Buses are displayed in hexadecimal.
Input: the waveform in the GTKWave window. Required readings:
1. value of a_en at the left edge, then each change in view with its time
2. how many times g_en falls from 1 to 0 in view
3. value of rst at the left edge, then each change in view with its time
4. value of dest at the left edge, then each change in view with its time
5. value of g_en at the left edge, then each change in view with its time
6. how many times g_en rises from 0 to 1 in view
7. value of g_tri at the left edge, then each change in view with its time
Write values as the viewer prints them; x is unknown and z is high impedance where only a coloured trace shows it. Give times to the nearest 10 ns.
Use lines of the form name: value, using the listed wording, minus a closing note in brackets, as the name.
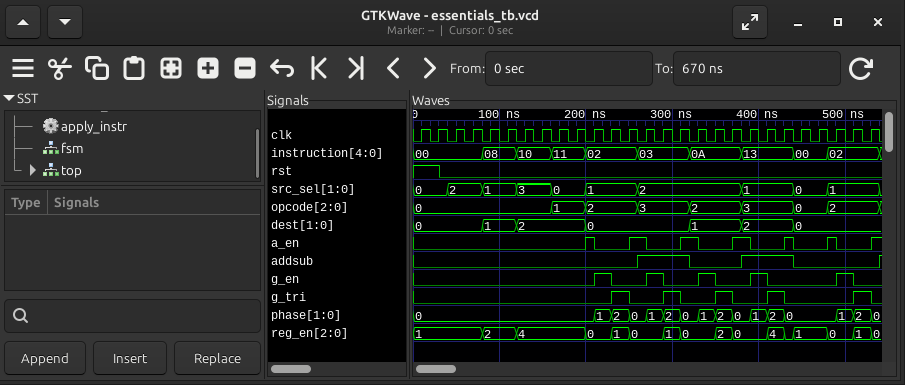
value of a_en at the left edge, then each change in view with its time: 0, 1 at 200 ns, 0 at 210 ns, 1 at 250 ns, 0 at 270 ns, 1 at 310 ns, 0 at 330 ns, 1 at 370 ns, 0 at 390 ns, 1 at 430 ns, 0 at 440 ns, 1 at 480 ns, 0 at 490 ns, 1 at 530 ns
how many times g_en falls from 1 to 0 in view: 5
value of rst at the left edge, then each change in view with its time: 1, 0 at 30 ns
value of dest at the left edge, then each change in view with its time: 0, 1 at 80 ns, 2 at 120 ns, 0 at 200 ns, 1 at 320 ns, 2 at 380 ns, 0 at 440 ns
value of g_en at the left edge, then each change in view with its time: 0, 1 at 210 ns, 0 at 230 ns, 1 at 270 ns, 0 at 290 ns, 1 at 330 ns, 0 at 350 ns, 1 at 390 ns, 0 at 410 ns, 1 at 490 ns, 0 at 510 ns
how many times g_en rises from 0 to 1 in view: 5
value of g_tri at the left edge, then each change in view with its time: 0, 1 at 230 ns, 0 at 250 ns, 1 at 290 ns, 0 at 310 ns, 1 at 350 ns, 0 at 370 ns, 1 at 410 ns, 0 at 430 ns, 1 at 510 ns, 0 at 530 ns
